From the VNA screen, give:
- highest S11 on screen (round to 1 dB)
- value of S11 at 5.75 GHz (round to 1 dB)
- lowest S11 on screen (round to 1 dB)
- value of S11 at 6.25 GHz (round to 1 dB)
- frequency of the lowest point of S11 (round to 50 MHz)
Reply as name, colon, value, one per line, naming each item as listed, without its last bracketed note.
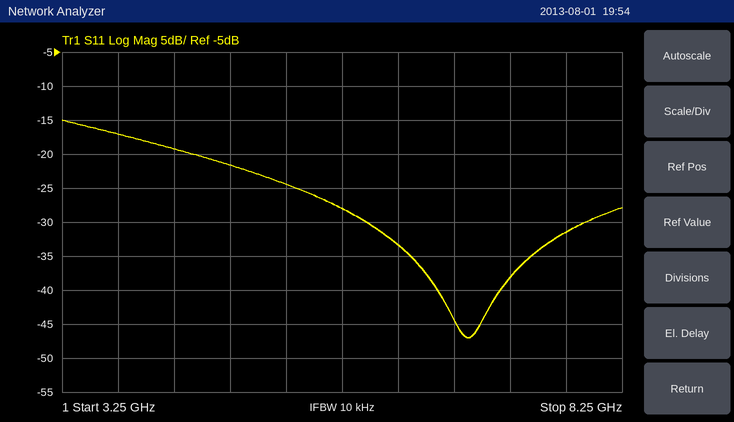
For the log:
highest S11 on screen: -15 dB
value of S11 at 5.75 GHz: -28 dB
lowest S11 on screen: -47 dB
value of S11 at 6.25 GHz: -33 dB
frequency of the lowest point of S11: 6.85 GHz
